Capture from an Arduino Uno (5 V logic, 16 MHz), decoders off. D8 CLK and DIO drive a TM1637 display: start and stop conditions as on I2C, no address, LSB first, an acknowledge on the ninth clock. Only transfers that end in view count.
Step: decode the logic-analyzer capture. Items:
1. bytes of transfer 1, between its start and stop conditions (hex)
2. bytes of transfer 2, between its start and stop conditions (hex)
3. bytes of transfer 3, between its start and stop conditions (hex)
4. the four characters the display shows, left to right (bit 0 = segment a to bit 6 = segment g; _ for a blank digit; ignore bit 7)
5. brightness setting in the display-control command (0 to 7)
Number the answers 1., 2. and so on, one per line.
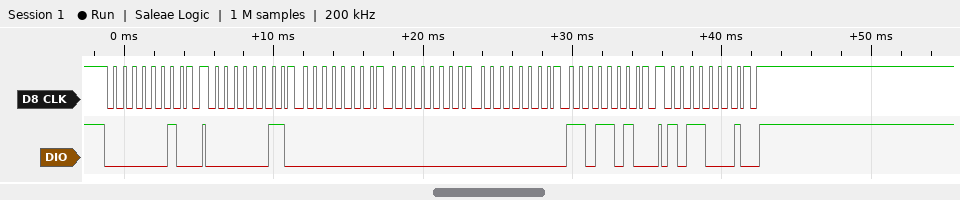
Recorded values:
1. 40
2. C0 00 00 00 5B
3. 8D
4. ___2
5. 5
